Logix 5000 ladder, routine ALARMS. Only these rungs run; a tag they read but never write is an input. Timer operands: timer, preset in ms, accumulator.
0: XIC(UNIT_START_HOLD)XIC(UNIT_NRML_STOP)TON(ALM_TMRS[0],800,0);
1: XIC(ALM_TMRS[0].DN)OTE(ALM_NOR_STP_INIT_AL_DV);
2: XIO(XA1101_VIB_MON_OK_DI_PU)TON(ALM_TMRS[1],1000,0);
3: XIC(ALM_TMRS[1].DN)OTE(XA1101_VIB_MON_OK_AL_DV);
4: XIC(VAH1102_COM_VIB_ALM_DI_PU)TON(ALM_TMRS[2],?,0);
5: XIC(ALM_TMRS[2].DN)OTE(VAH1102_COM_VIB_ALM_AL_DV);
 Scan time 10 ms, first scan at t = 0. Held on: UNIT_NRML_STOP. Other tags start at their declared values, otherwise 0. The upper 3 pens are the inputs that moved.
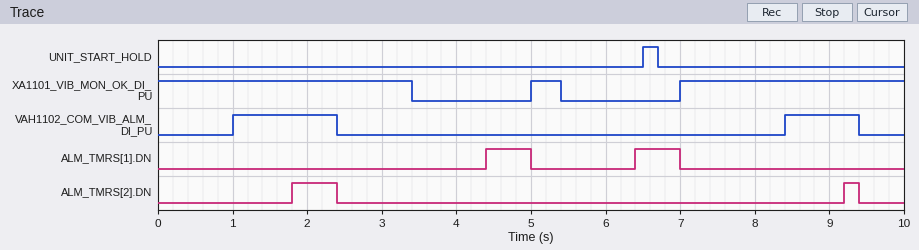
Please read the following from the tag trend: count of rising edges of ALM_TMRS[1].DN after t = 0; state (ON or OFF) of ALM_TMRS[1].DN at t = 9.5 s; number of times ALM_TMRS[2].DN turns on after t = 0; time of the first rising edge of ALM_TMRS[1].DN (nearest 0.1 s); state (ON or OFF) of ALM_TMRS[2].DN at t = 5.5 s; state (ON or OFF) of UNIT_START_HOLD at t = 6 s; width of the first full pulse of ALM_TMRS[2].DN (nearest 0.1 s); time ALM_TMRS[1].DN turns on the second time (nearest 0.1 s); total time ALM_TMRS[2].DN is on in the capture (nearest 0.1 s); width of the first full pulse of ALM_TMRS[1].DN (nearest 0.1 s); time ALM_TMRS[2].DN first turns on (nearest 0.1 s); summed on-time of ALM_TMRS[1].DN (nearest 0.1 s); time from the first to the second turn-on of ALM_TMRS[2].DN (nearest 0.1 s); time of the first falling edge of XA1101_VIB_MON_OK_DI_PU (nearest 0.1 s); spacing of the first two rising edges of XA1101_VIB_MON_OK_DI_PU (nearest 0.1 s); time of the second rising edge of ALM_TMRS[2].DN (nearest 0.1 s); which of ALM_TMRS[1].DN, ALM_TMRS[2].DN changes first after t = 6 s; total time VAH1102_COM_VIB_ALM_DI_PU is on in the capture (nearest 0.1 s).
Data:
2
OFF
2
4.4 s
OFF
OFF
0.6 s
6.4 s
0.8 s
0.6 s
1.8 s
1.2 s
7.4 s
3.4 s
2.0 s
9.2 s
ALM_TMRS[1].DN
2.4 s
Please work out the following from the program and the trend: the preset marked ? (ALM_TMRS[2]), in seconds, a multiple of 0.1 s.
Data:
0.8 s
